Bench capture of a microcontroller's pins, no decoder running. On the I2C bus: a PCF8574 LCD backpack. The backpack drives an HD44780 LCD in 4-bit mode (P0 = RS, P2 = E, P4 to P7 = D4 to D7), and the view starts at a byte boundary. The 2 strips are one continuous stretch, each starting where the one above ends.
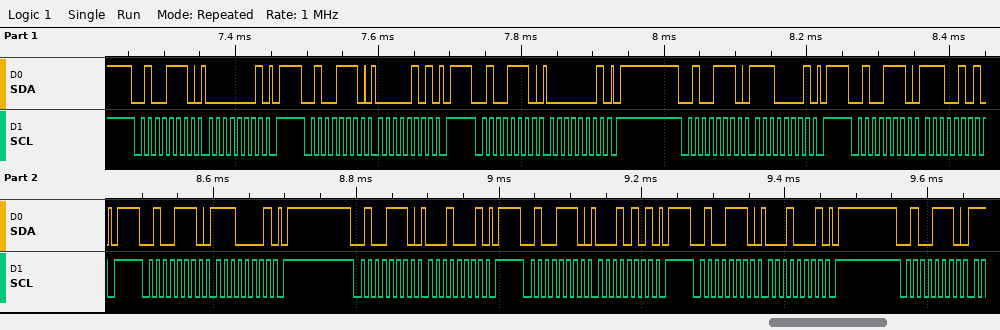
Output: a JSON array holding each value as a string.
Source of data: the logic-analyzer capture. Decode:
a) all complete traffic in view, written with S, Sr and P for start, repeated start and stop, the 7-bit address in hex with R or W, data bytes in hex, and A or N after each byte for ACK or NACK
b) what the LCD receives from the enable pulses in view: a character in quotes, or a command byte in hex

["S 27W A 01 A P S 27W A 05 A P S 27W A 01 A P S 27W A E1 A P S 27W A E5 A P S 27W A E1 A P S 27W A 11 A P S 27W A 15 A P S 27W A 11 A P S 27W A", "data 0x0E"]
